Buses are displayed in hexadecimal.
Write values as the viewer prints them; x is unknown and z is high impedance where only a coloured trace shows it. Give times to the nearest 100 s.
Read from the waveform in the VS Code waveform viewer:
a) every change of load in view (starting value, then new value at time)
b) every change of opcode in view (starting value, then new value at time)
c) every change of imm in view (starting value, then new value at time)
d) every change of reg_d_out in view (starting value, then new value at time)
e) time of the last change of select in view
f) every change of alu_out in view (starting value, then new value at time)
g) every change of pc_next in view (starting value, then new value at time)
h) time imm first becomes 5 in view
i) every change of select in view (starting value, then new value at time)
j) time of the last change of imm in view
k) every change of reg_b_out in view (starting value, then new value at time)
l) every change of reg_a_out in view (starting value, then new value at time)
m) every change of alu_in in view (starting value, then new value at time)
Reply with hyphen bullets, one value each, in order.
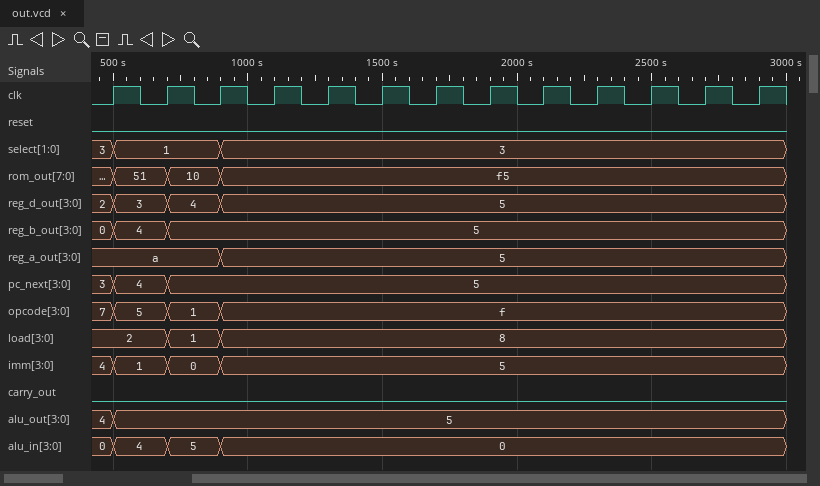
- 2, 1 at 700 s, 8 at 900 s
- 7, 5 at 500 s, 1 at 700 s, f at 900 s
- 4, 1 at 500 s, 0 at 700 s, 5 at 900 s
- 2, 3 at 500 s, 4 at 700 s, 5 at 900 s
- 900 s
- 4, 5 at 500 s
- 3, 4 at 500 s, 5 at 700 s
- 900 s
- 3, 1 at 500 s, 3 at 900 s
- 900 s
- 0, 4 at 500 s, 5 at 700 s
- a, 5 at 900 s
- 0, 4 at 500 s, 5 at 700 s, 0 at 900 s
